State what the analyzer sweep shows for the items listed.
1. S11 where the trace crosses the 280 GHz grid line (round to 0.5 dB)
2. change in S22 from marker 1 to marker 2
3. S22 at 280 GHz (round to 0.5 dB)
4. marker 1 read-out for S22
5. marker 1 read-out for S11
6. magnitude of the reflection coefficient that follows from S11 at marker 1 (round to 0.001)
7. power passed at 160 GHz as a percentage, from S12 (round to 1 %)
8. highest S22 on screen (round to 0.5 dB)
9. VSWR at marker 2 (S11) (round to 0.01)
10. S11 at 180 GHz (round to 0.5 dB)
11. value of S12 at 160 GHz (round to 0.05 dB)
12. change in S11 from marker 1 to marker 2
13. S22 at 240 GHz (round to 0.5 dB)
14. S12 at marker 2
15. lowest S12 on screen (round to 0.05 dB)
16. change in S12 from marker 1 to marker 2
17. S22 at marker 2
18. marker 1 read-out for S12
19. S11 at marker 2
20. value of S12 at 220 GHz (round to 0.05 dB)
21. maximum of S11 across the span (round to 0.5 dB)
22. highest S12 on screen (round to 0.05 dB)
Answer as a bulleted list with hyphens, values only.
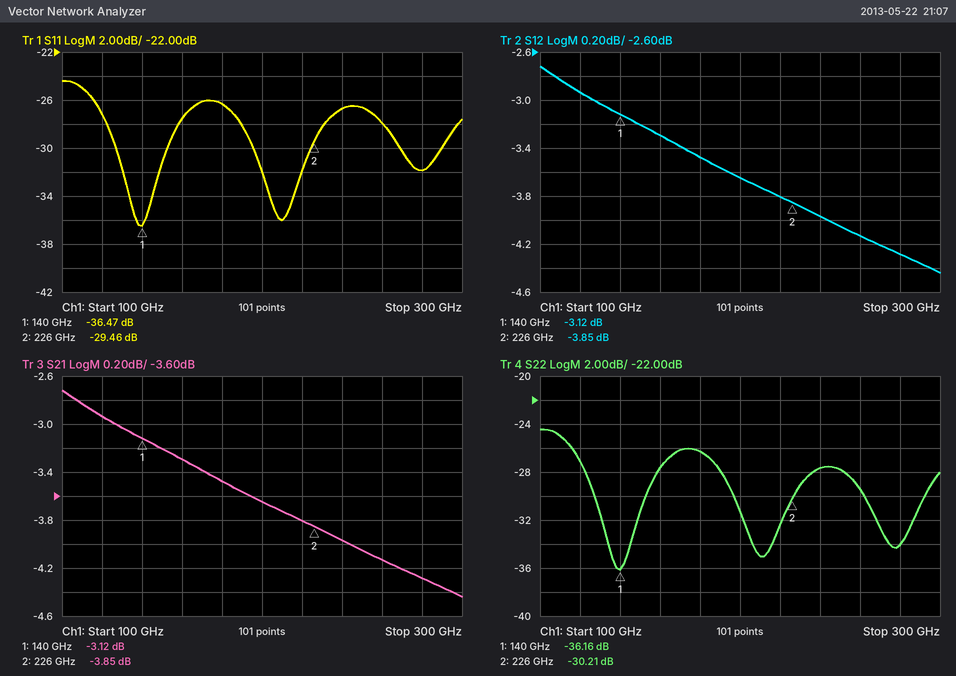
- -32.0 dB
- 5.95 dB
- -34.0 dB
- -36.16 dB
- -36.47 dB
- 0.015
- 47 %
- -24.5 dB
- 1.07
- -26.5 dB
- -3.30 dB
- 7.01 dB
- -27.5 dB
- -3.85 dB
- -4.45 dB
- -0.73 dB
- -30.21 dB
- -3.12 dB
- -29.46 dB
- -3.80 dB
- -24.5 dB
- -2.70 dB
